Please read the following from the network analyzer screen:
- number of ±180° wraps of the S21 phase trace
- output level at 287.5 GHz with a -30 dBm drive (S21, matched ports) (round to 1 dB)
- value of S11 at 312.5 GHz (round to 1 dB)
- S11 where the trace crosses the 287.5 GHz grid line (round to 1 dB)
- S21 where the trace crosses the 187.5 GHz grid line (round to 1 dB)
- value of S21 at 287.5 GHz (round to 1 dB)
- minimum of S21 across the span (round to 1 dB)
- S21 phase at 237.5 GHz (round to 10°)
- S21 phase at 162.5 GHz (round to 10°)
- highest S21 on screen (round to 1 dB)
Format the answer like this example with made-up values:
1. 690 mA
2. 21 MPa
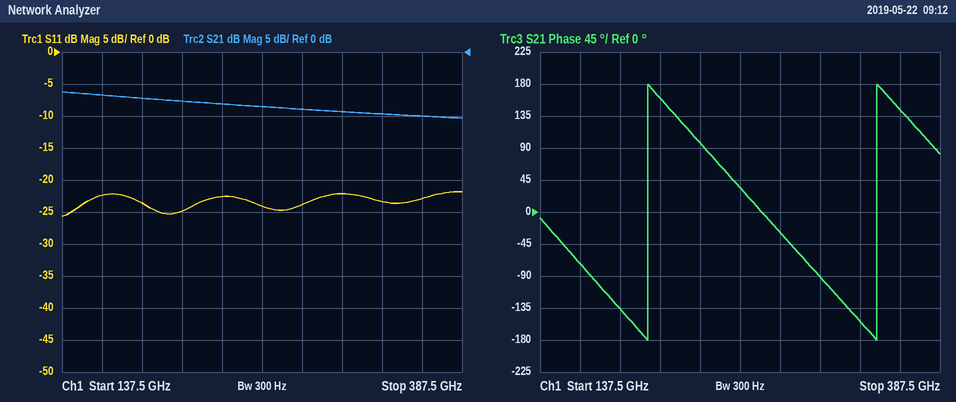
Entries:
1. 2
2. -39 dBm
3. -22 dB
4. -24 dB
5. -7 dB
6. -9 dB
7. -10 dB
8. 100°
9. -70°
10. -6 dB
